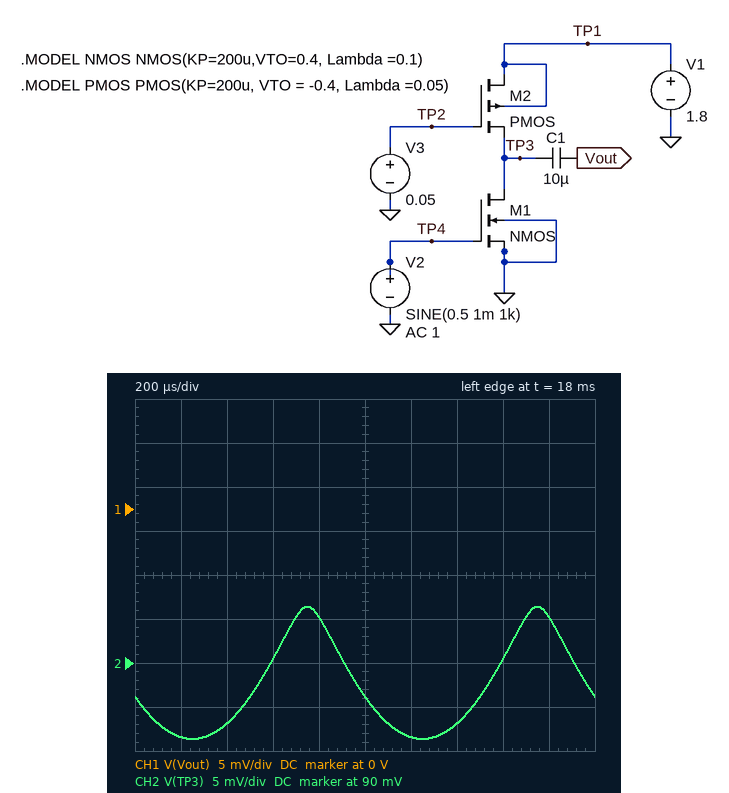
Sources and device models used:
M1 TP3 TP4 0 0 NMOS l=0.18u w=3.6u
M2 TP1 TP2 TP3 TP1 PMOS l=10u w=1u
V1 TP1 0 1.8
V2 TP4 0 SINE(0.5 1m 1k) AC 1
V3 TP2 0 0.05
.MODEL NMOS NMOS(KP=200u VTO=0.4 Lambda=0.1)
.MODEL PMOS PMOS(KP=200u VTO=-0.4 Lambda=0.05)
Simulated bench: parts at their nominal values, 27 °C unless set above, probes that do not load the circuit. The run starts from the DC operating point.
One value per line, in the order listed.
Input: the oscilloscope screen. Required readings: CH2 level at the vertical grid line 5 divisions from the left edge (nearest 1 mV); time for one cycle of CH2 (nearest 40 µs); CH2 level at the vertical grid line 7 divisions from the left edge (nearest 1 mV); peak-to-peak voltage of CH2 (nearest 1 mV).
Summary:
86 mV
1.00 ms
83 mV
15 mV
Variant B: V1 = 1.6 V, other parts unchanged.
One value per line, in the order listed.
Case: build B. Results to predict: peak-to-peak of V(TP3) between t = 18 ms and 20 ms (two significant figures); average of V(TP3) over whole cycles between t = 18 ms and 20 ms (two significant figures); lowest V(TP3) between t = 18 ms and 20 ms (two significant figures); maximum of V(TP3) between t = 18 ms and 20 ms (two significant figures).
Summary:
1.7 mV
46 mV
45 mV
47 mV
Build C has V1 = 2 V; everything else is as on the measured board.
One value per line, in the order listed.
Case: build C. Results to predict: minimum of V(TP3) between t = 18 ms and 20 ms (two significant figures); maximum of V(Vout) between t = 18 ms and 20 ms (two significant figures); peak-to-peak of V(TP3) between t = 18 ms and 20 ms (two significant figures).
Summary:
970 mV
1.0 V
60 mV
